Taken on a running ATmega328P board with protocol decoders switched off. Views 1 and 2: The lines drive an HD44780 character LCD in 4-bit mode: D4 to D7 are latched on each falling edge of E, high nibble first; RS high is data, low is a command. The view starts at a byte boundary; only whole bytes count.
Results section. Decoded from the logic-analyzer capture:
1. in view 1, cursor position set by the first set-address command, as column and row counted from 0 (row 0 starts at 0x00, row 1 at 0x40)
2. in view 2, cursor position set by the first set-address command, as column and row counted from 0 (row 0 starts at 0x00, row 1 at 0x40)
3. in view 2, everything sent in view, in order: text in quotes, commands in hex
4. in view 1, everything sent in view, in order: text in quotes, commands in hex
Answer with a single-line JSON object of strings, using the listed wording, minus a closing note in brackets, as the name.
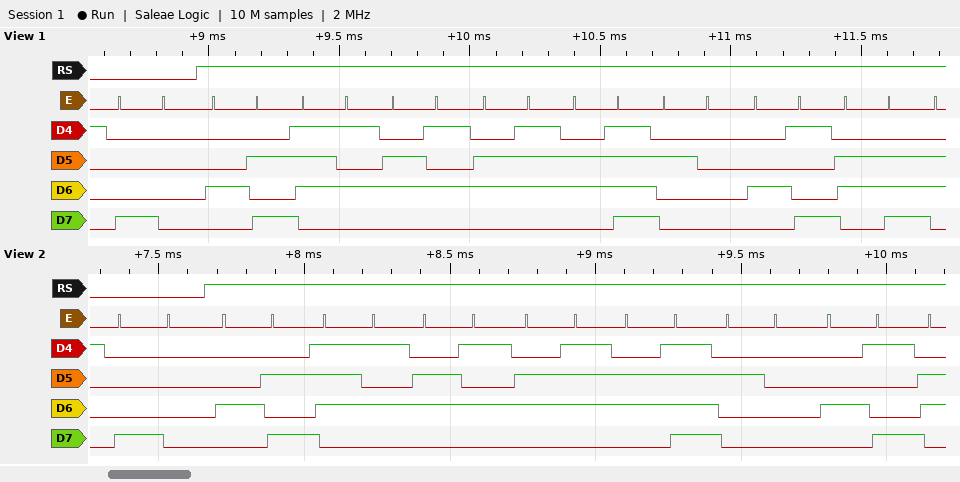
{"in view 1, cursor position set by the first set-address command, as column and row counted from 0": "column 0, row 0", "in view 2, cursor position set by the first set-address command, as column and row counted from 0": "column 0, row 0", "in view 2, everything sent in view, in order: text in quotes, commands in hex": "0x80 \"Juego I\"", "in view 1, everything sent in view, in order: text in quotes, commands in hex": "0x80 \"Juego In\""}
